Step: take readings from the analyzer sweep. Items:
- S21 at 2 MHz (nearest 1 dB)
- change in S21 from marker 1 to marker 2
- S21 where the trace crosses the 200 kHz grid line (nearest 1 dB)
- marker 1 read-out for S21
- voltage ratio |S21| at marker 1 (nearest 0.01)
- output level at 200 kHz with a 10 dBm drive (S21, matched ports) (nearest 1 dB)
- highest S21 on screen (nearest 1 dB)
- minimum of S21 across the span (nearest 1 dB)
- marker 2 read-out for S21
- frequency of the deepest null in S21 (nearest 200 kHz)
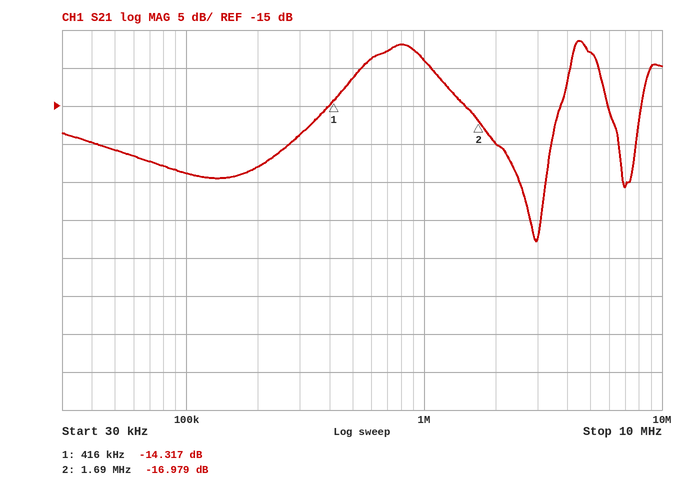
-20 dB
-2.662 dB
-23 dB
-14.317 dB
0.19
-13 dBm
-6 dB
-33 dB
-16.979 dB
3.0 MHz
